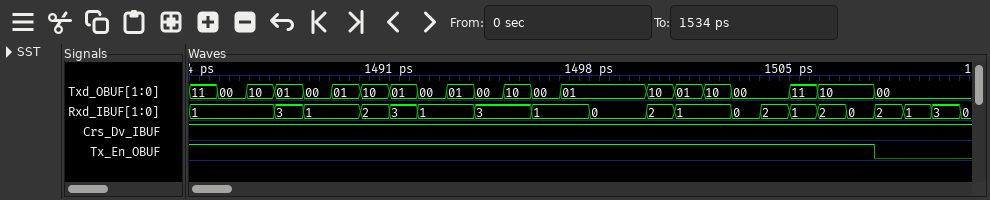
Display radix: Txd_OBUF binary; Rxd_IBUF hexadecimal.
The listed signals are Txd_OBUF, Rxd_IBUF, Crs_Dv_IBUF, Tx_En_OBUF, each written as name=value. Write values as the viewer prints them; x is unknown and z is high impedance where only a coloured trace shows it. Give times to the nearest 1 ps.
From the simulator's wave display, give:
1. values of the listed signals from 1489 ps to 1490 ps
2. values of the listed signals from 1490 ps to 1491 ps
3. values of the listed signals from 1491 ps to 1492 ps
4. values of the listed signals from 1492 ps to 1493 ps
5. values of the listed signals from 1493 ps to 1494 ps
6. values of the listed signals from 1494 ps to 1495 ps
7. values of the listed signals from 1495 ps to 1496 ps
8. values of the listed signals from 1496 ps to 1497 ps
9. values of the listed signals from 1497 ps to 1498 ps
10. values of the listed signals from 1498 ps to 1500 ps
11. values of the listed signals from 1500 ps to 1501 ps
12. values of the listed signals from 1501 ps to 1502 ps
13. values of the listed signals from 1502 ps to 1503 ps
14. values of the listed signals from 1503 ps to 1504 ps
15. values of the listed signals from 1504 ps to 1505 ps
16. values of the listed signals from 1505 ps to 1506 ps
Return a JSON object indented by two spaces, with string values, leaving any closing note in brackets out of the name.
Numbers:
{
  "values of the listed signals from 1489 ps to 1490 ps": "Txd_OBUF=01, Rxd_IBUF=1, Crs_Dv_IBUF=1, Tx_En_OBUF=1",
  "values of the listed signals from 1490 ps to 1491 ps": "Txd_OBUF=10, Rxd_IBUF=2, Crs_Dv_IBUF=1, Tx_En_OBUF=1",
  "values of the listed signals from 1491 ps to 1492 ps": "Txd_OBUF=01, Rxd_IBUF=3, Crs_Dv_IBUF=1, Tx_En_OBUF=1",
  "values of the listed signals from 1492 ps to 1493 ps": "Txd_OBUF=00, Rxd_IBUF=1, Crs_Dv_IBUF=1, Tx_En_OBUF=1",
  "values of the listed signals from 1493 ps to 1494 ps": "Txd_OBUF=01, Rxd_IBUF=1, Crs_Dv_IBUF=1, Tx_En_OBUF=1",
  "values of the listed signals from 1494 ps to 1495 ps": "Txd_OBUF=00, Rxd_IBUF=3, Crs_Dv_IBUF=1, Tx_En_OBUF=1",
  "values of the listed signals from 1495 ps to 1496 ps": "Txd_OBUF=10, Rxd_IBUF=3, Crs_Dv_IBUF=1, Tx_En_OBUF=1",
  "values of the listed signals from 1496 ps to 1497 ps": "Txd_OBUF=00, Rxd_IBUF=1, Crs_Dv_IBUF=1, Tx_En_OBUF=1",
  "values of the listed signals from 1497 ps to 1498 ps": "Txd_OBUF=01, Rxd_IBUF=1, Crs_Dv_IBUF=1, Tx_En_OBUF=1",
  "values of the listed signals from 1498 ps to 1500 ps": "Txd_OBUF=01, Rxd_IBUF=0, Crs_Dv_IBUF=1, Tx_En_OBUF=1",
  "values of the listed signals from 1500 ps to 1501 ps": "Txd_OBUF=10, Rxd_IBUF=2, Crs_Dv_IBUF=1, Tx_En_OBUF=1",
  "values of the listed signals from 1501 ps to 1502 ps": "Txd_OBUF=01, Rxd_IBUF=1, Crs_Dv_IBUF=1, Tx_En_OBUF=1",
  "values of the listed signals from 1502 ps to 1503 ps": "Txd_OBUF=10, Rxd_IBUF=1, Crs_Dv_IBUF=1, Tx_En_OBUF=1",
  "values of the listed signals from 1503 ps to 1504 ps": "Txd_OBUF=00, Rxd_IBUF=0, Crs_Dv_IBUF=1, Tx_En_OBUF=1",
  "values of the listed signals from 1504 ps to 1505 ps": "Txd_OBUF=00, Rxd_IBUF=2, Crs_Dv_IBUF=1, Tx_En_OBUF=1",
  "values of the listed signals from 1505 ps to 1506 ps": "Txd_OBUF=11, Rxd_IBUF=1, Crs_Dv_IBUF=1, Tx_En_OBUF=1"
}
